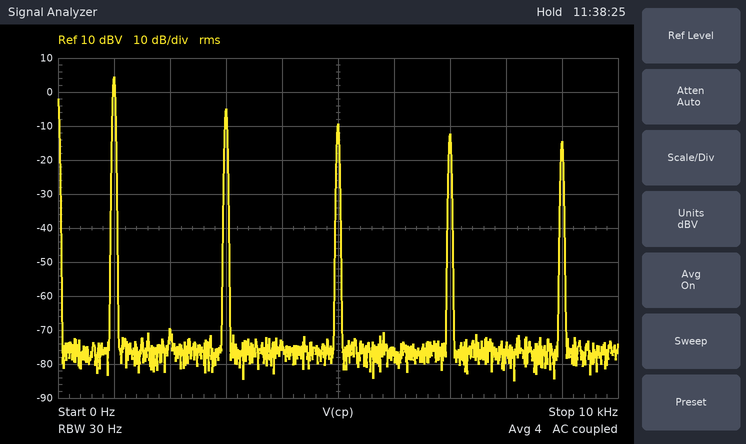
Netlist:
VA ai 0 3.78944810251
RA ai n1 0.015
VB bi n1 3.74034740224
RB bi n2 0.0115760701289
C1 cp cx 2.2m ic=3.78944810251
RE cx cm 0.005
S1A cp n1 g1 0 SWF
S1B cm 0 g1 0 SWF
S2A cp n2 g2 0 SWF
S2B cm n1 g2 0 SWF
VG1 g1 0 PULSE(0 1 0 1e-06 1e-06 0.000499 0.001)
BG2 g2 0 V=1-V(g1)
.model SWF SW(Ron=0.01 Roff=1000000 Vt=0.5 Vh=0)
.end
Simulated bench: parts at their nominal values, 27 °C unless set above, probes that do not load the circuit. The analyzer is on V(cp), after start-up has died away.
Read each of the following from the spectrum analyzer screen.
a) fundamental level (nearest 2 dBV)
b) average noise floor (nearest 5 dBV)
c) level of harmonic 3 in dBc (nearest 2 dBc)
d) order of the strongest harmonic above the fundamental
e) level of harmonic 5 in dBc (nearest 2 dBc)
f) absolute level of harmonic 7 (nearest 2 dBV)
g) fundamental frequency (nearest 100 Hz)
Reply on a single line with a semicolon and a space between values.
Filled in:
4 dBV; -75 dBV; -10 dBc; 3; -14 dBc; -12 dBV; 1.0 kHz
